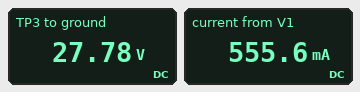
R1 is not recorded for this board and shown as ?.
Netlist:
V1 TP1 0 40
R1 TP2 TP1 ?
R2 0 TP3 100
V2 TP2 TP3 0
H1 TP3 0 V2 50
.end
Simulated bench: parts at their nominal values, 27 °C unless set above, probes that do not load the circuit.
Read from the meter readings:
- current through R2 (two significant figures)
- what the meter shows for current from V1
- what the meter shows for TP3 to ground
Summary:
280 mA
555.6 mA
27.78 V
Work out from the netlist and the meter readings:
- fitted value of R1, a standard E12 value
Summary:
22 Ω
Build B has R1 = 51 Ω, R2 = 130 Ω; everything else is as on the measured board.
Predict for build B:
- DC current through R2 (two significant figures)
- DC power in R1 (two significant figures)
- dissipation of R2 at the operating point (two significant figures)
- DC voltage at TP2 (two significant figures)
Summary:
150 mA
8.0 W
3.0 W
20 V
